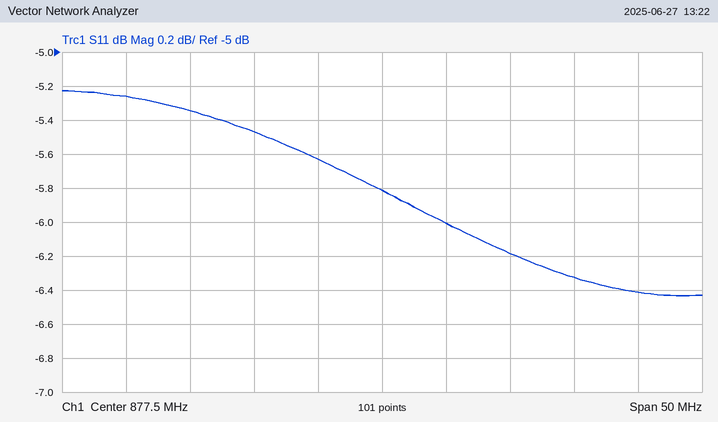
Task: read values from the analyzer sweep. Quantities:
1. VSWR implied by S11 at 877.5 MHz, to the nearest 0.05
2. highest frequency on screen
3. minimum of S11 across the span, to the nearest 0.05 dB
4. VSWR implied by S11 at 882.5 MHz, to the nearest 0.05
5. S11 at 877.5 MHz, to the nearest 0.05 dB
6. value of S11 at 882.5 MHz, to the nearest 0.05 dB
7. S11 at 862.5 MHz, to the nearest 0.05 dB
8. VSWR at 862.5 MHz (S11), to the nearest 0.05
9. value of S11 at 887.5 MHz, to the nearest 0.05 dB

3.10
902.5 MHz
-6.45 dB
3.00
-5.80 dB
-6.00 dB
-5.35 dB
3.35
-6.20 dB
